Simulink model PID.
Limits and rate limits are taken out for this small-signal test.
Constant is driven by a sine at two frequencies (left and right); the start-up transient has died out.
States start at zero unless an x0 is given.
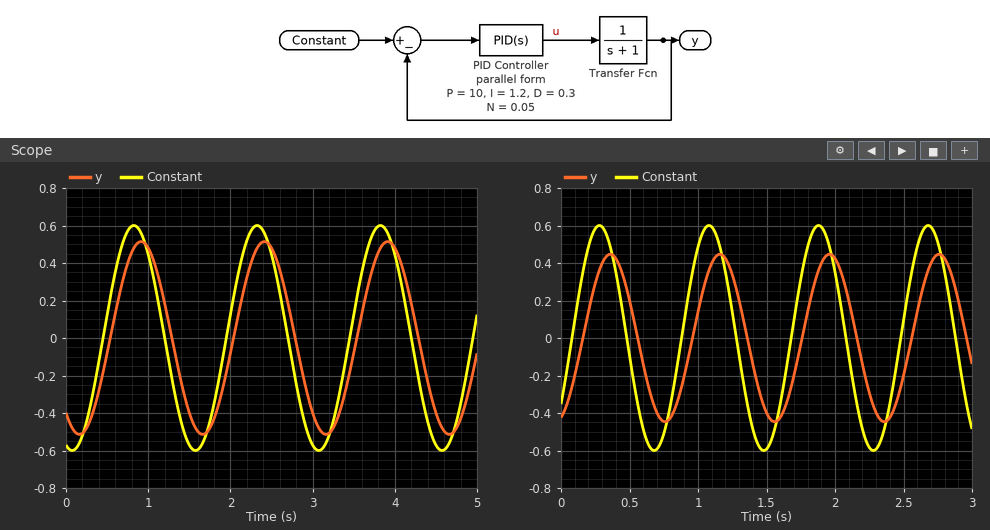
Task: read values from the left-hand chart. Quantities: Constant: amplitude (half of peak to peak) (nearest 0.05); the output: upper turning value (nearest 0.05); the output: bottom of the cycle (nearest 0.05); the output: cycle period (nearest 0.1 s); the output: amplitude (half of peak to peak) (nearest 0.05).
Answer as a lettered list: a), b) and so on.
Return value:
a) 0.60
b) 0.50
c) -0.50
d) 1.5 s
e) 0.50
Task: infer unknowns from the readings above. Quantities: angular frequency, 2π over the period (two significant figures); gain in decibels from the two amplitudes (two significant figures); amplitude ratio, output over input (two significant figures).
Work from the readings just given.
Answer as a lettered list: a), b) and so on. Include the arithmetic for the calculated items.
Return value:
a) 2π / 1.5 = 4.2 rad/s
b) 20 log10(0.5 / 0.6) = -1.6 dB
c) 0.5 / 0.6 = 0.83
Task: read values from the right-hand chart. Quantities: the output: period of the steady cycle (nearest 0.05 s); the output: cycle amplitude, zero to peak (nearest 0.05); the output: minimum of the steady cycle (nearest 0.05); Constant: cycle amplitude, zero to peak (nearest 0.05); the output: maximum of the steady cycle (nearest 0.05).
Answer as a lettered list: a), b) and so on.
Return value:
a) 0.80 s
b) 0.45
c) -0.45
d) 0.60
e) 0.45
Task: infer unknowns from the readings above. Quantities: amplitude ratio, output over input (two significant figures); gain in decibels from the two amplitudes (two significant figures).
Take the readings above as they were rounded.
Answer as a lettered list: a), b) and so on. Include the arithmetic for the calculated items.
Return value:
a) 0.45 / 0.6 = 0.75
b) 20 log10(0.45 / 0.6) = -2.5 dB
